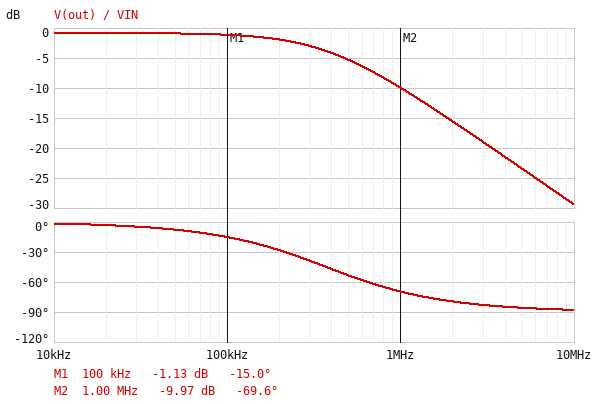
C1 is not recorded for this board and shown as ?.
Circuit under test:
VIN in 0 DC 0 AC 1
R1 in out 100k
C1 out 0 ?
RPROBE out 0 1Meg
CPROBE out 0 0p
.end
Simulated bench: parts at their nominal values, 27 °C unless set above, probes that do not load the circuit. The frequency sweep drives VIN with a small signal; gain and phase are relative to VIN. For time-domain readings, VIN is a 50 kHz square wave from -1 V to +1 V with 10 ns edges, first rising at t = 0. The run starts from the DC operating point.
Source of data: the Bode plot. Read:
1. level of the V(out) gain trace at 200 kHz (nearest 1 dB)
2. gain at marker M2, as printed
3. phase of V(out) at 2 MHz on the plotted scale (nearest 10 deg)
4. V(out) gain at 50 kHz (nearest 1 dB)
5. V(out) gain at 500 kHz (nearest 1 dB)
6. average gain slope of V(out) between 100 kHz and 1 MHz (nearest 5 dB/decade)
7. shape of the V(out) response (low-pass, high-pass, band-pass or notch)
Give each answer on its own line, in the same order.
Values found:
-2 dB
-9.97 dB
-80 deg
-1 dB
-5 dB
-10 dB/decade
low-pass
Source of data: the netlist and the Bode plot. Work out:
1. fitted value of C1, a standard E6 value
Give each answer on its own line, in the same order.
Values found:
4.7 pF
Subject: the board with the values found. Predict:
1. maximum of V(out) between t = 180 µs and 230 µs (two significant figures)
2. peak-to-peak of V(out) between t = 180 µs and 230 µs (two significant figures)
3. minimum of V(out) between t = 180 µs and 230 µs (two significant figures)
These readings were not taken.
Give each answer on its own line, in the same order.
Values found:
910 mV
1.8 V
-910 mV
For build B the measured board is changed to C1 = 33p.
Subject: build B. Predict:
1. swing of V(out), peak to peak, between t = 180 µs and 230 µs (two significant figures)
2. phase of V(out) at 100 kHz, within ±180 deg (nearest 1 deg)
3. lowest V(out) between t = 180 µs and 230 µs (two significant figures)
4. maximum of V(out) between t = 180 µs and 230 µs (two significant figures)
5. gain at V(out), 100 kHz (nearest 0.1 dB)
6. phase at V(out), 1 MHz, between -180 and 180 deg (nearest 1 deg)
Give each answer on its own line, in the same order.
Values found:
1.7 V
-62 deg
-850 mV
850 mV
-7.4 dB
-87 deg
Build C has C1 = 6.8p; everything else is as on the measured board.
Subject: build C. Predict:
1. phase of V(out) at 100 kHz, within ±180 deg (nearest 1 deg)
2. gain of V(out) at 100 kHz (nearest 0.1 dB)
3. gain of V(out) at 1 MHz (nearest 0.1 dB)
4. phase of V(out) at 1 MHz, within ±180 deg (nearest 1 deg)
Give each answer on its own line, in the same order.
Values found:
-21 deg
-1.4 dB
-12.9 dB
-76 deg
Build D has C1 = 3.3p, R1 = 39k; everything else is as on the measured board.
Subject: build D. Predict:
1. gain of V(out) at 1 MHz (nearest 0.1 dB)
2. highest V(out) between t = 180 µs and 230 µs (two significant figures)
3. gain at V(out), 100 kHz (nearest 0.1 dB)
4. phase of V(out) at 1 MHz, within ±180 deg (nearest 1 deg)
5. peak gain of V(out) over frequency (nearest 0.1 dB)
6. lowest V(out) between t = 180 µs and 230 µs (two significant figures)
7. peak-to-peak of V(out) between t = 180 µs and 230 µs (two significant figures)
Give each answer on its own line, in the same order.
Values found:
-2.4 dB
960 mV
-0.4 dB
-38 deg
-0.3 dB
-960 mV
1.9 V
